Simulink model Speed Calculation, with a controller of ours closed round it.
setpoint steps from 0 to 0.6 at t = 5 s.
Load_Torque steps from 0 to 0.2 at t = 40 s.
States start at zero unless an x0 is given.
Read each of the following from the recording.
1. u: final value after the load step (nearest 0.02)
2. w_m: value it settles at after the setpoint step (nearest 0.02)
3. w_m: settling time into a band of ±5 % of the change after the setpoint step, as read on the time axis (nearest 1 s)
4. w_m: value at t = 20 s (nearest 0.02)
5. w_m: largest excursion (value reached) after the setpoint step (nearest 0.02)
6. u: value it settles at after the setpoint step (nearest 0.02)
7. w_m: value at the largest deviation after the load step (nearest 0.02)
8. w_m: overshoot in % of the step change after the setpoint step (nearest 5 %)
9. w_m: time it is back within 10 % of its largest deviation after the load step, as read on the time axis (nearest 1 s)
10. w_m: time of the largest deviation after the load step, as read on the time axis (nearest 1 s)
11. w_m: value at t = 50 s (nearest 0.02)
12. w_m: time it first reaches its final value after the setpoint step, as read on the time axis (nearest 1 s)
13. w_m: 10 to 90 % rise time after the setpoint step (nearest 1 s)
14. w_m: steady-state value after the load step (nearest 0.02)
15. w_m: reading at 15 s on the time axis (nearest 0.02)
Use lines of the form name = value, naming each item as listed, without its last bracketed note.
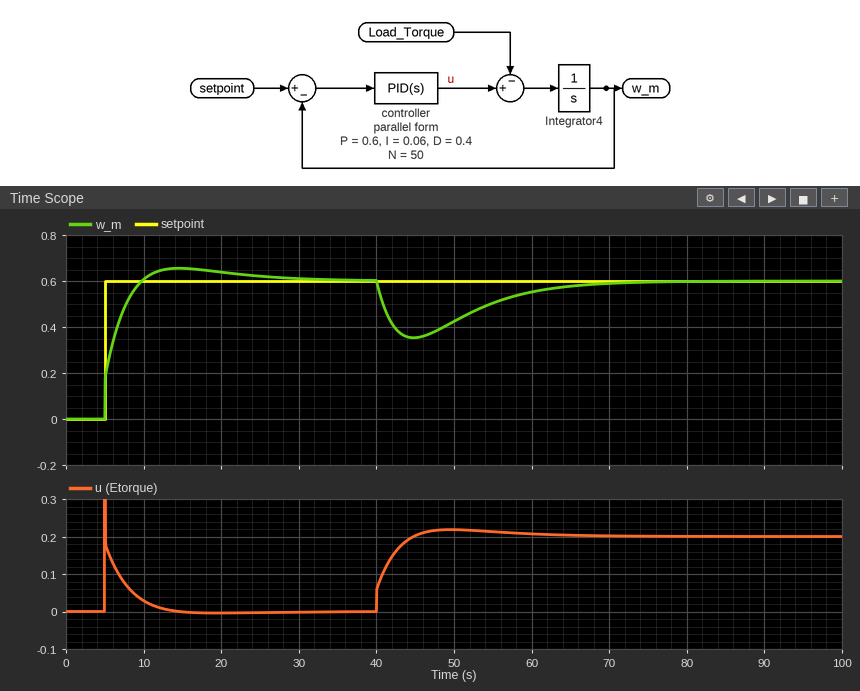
u: final value after the load step = 0.20
w_m: value it settles at after the setpoint step = 0.60
w_m: settling time into a band of ±5 % of the change after the setpoint step, as read on the time axis = 22 s
w_m: value at t = 20 s = 0.64
w_m: largest excursion (value reached) after the setpoint step = 0.66
u: value it settles at after the setpoint step = 0.00
w_m: value at the largest deviation after the load step = 0.36
w_m: overshoot in % of the step change after the setpoint step = 10 %
w_m: time it is back within 10 % of its largest deviation after the load step, as read on the time axis = 64 s
w_m: time of the largest deviation after the load step, as read on the time axis = 45 s
w_m: value at t = 50 s = 0.42
w_m: time it first reaches its final value after the setpoint step, as read on the time axis = 10 s
w_m: 10 to 90 % rise time after the setpoint step = 3 s
w_m: steady-state value after the load step = 0.60
w_m: reading at 15 s on the time axis = 0.66
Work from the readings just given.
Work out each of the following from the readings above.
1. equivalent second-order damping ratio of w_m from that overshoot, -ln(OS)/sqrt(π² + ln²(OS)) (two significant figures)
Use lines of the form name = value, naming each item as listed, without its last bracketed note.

equivalent second-order damping ratio of w_m from that overshoot, -ln(OS)/sqrt(π² + ln²(OS)) = 0.59
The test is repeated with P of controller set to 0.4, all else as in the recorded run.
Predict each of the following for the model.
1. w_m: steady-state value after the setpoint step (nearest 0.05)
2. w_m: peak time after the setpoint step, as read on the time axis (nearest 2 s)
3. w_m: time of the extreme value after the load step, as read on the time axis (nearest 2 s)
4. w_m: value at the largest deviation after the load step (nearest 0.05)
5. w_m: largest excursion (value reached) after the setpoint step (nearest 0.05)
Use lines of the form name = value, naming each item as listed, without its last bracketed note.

w_m: steady-state value after the setpoint step = 0.60
w_m: peak time after the setpoint step, as read on the time axis = 16 s
w_m: time of the extreme value after the load step, as read on the time axis = 46 s
w_m: value at the largest deviation after the load step = 0.30
w_m: largest excursion (value reached) after the setpoint step = 0.70
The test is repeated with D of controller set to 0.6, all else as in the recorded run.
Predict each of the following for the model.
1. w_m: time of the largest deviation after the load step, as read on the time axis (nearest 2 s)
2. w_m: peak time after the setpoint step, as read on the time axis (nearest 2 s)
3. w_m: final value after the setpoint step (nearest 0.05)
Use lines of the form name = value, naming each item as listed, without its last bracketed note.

w_m: time of the largest deviation after the load step, as read on the time axis = 46 s
w_m: peak time after the setpoint step, as read on the time axis = 16 s
w_m: final value after the setpoint step = 0.60
